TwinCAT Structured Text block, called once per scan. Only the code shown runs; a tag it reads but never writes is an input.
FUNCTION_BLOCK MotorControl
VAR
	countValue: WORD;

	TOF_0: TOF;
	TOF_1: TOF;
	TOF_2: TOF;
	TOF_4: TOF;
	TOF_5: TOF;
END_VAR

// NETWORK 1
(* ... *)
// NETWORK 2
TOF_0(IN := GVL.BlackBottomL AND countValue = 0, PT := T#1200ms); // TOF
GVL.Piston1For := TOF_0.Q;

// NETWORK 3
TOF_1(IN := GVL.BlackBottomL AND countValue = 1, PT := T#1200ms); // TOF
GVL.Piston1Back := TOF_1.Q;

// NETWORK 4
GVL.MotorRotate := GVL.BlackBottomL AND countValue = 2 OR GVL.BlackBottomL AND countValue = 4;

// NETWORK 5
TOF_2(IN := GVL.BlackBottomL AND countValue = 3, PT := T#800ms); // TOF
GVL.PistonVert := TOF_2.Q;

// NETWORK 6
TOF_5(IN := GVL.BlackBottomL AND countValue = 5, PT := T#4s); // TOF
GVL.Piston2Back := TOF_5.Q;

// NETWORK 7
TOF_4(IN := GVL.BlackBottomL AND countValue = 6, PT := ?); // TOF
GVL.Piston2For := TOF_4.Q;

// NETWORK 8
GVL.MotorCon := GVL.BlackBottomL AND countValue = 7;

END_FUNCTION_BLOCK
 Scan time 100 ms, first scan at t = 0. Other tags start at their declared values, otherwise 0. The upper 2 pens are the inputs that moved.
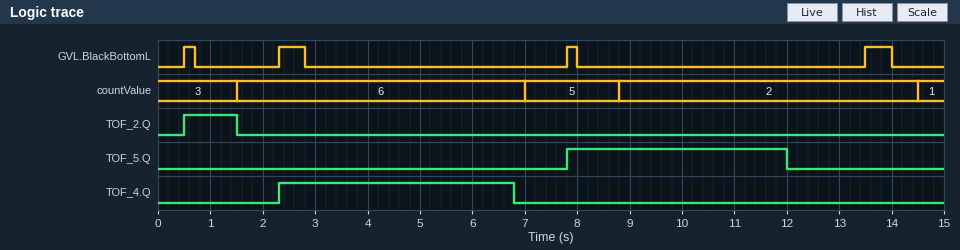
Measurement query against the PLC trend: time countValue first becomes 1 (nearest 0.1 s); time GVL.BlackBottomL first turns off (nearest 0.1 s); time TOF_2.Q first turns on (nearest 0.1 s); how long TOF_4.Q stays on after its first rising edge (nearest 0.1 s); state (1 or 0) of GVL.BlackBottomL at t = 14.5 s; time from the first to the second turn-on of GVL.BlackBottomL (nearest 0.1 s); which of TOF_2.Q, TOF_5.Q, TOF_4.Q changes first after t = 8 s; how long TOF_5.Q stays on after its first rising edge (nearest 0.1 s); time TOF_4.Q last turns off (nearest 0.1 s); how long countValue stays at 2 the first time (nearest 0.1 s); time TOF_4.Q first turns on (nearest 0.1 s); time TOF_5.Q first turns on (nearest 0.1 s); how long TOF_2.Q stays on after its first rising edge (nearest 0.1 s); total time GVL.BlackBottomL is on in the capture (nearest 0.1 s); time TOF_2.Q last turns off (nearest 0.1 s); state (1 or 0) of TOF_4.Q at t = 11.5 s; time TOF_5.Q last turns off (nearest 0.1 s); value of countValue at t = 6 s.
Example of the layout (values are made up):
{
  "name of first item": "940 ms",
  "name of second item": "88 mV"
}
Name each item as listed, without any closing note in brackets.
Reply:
{
  "time countValue first becomes 1": "14.5 s",
  "time GVL.BlackBottomL first turns off": "0.7 s",
  "time TOF_2.Q first turns on": "0.5 s",
  "how long TOF_4.Q stays on after its first rising edge": "4.5 s",
  "state (1 or 0) of GVL.BlackBottomL at t = 14.5 s": "0",
  "time from the first to the second turn-on of GVL.BlackBottomL": "1.8 s",
  "which of TOF_2.Q, TOF_5.Q, TOF_4.Q changes first after t = 8 s": "TOF_5.Q",
  "how long TOF_5.Q stays on after its first rising edge": "4.2 s",
  "time TOF_4.Q last turns off": "6.8 s",
  "how long countValue stays at 2 the first time": "5.7 s",
  "time TOF_4.Q first turns on": "2.3 s",
  "time TOF_5.Q first turns on": "7.8 s",
  "how long TOF_2.Q stays on after its first rising edge": "1.0 s",
  "total time GVL.BlackBottomL is on in the capture": "1.4 s",
  "time TOF_2.Q last turns off": "1.5 s",
  "state (1 or 0) of TOF_4.Q at t = 11.5 s": "0",
  "time TOF_5.Q last turns off": "12.0 s",
  "value of countValue at t = 6 s": "6"
}
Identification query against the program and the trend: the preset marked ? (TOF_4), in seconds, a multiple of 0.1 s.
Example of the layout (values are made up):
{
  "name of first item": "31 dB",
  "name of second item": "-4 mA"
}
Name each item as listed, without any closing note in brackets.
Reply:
{
  "the preset marked ? (TOF_4), in seconds, a multiple of 0.1 s": "4.0 s"
}
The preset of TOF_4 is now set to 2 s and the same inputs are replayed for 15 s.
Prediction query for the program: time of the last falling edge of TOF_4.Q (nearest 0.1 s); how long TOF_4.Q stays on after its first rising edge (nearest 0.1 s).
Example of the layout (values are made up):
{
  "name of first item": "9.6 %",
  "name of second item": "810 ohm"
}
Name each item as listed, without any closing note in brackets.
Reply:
{
  "time of the last falling edge of TOF_4.Q": "4.8 s",
  "how long TOF_4.Q stays on after its first rising edge": "2.5 s"
}
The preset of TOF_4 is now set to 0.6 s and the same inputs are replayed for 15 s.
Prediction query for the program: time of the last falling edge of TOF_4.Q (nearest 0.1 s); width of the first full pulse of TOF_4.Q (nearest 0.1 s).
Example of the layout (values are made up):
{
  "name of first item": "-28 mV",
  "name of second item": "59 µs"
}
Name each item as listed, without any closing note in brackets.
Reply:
{
  "time of the last falling edge of TOF_4.Q": "3.4 s",
  "width of the first full pulse of TOF_4.Q": "1.1 s"
}
